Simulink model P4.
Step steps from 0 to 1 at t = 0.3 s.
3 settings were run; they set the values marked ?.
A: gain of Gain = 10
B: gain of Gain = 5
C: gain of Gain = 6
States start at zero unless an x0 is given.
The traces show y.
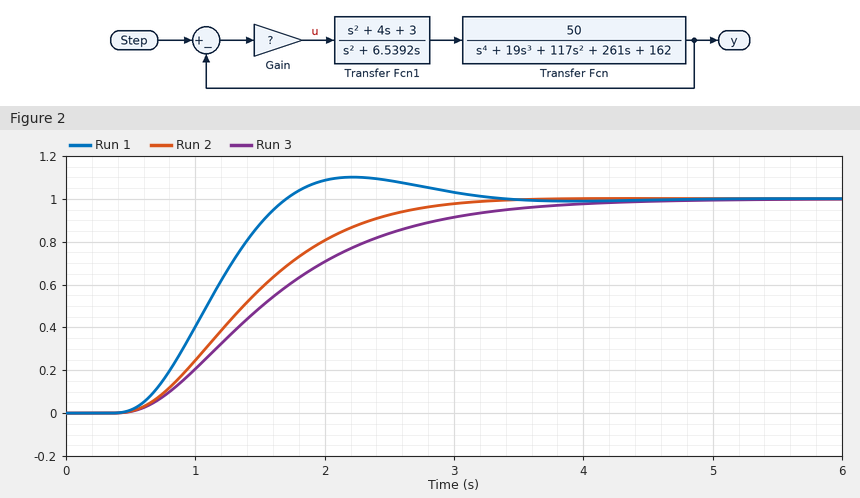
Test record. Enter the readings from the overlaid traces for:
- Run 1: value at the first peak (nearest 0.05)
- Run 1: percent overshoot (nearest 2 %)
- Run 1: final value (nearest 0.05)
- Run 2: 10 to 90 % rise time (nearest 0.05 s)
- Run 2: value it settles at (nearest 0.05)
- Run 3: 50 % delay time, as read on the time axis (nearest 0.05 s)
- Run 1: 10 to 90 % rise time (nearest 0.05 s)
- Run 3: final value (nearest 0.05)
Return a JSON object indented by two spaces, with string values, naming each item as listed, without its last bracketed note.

{
  "Run 1: value at the first peak": "1.10",
  "Run 1: percent overshoot": "10 %",
  "Run 1: final value": "1.00",
  "Run 2: 10 to 90 % rise time": "1.60 s",
  "Run 2: value it settles at": "1.00",
  "Run 3: 50 % delay time, as read on the time axis": "1.50 s",
  "Run 1: 10 to 90 % rise time": "0.85 s",
  "Run 3: final value": "1.00"
}
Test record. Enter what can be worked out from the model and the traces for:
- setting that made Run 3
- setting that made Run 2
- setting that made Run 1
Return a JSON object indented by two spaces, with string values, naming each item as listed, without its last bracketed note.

{
  "setting that made Run 3": "B",
  "setting that made Run 2": "C",
  "setting that made Run 1": "A"
}
